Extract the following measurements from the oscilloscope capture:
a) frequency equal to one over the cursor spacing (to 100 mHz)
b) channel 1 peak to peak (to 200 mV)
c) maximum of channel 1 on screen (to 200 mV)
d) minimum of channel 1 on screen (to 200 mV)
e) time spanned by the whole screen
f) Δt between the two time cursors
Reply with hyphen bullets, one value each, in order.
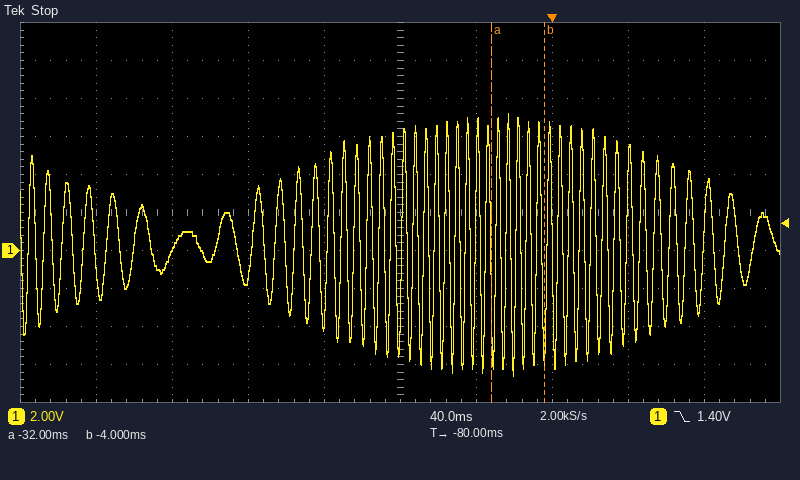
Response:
- 35.7 Hz
- 13.8 V
- 7.2 V
- -6.6 V
- 400 ms
- 28 ms
